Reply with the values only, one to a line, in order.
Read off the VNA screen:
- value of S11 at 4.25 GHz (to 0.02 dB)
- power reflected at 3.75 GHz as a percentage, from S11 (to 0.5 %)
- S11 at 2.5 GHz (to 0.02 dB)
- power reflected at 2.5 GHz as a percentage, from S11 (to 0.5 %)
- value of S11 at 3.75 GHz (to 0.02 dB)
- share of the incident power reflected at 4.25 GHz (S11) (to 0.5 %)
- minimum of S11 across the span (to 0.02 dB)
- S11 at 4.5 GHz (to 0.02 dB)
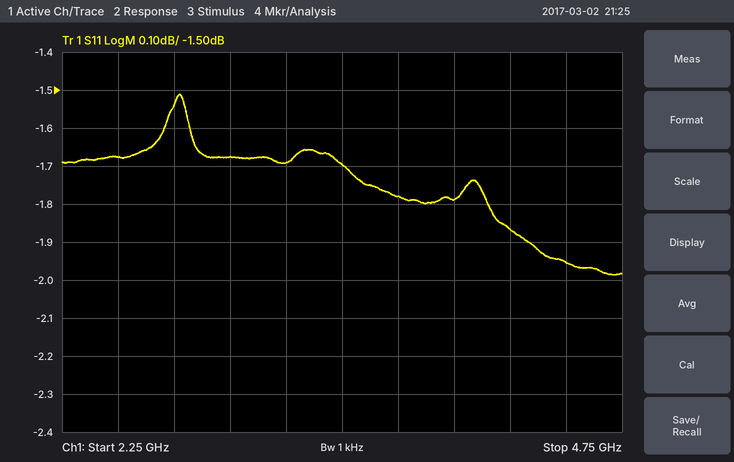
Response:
-1.86 dB
66.5 %
-1.68 dB
68.0 %
-1.78 dB
65.0 %
-1.98 dB
-1.96 dB
